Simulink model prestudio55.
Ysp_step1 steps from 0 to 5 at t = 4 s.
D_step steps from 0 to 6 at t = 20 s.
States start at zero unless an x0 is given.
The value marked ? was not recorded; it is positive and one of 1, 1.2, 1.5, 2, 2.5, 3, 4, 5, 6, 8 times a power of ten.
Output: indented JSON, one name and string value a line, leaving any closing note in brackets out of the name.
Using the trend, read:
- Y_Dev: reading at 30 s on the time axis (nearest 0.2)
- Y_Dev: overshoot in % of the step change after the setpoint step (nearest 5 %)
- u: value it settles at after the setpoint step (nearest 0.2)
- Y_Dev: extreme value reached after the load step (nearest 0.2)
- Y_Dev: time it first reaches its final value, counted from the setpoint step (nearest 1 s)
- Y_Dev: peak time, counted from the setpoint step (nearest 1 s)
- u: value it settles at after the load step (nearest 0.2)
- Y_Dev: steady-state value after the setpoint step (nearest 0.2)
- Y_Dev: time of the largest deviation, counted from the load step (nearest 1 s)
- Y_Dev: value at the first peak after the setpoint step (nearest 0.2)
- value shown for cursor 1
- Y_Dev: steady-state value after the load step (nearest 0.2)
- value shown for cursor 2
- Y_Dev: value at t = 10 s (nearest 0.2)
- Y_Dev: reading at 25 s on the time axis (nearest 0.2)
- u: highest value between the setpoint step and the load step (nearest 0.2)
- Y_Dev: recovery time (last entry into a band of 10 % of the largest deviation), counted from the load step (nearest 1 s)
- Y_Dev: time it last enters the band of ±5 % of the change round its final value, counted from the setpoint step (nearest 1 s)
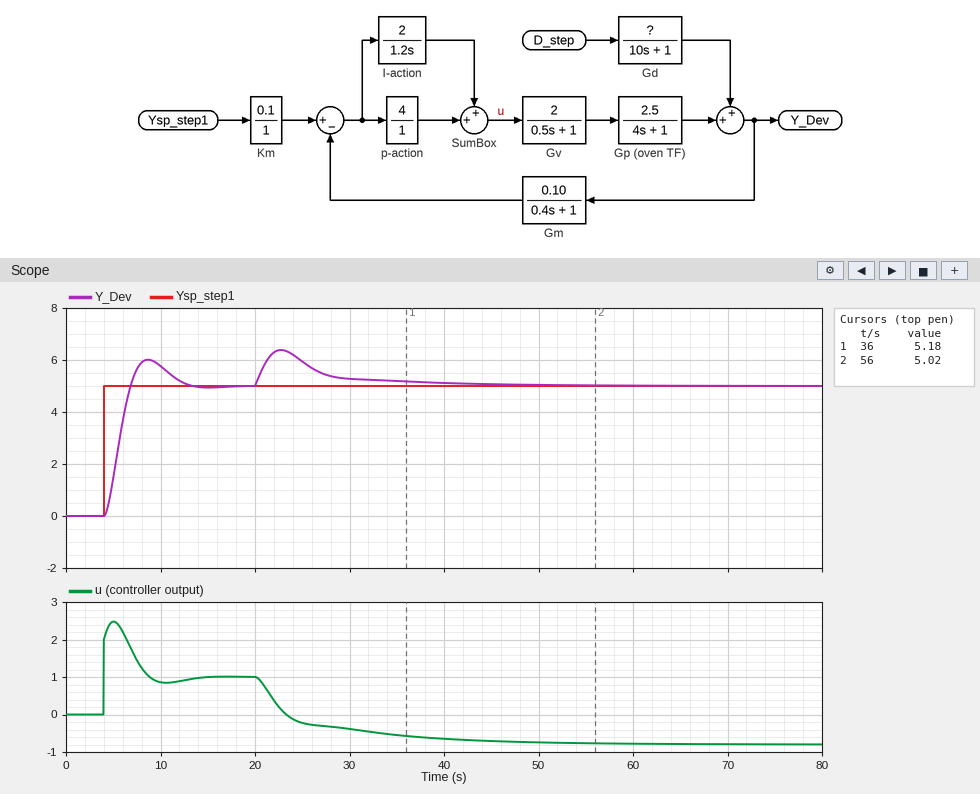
{
  "Y_Dev: reading at 30 s on the time axis": "5.2",
  "Y_Dev: overshoot in % of the step change after the setpoint step": "20 %",
  "u: value it settles at after the setpoint step": "1.0",
  "Y_Dev: extreme value reached after the load step": "6.4",
  "Y_Dev: time it first reaches its final value, counted from the setpoint step": "3 s",
  "Y_Dev: peak time, counted from the setpoint step": "5 s",
  "u: value it settles at after the load step": "-0.8",
  "Y_Dev: steady-state value after the setpoint step": "5.0",
  "Y_Dev: time of the largest deviation, counted from the load step": "3 s",
  "Y_Dev: value at the first peak after the setpoint step": "6.0",
  "value shown for cursor 1": "5.18",
  "Y_Dev: steady-state value after the load step": "5.0",
  "value shown for cursor 2": "5.02",
  "Y_Dev: value at t = 10 s": "5.8",
  "Y_Dev: reading at 25 s on the time axis": "6.0",
  "u: highest value between the setpoint step and the load step": "2.4",
  "Y_Dev: recovery time (last entry into a band of 10 % of the largest deviation), counted from the load step": "18 s",
  "Y_Dev: time it last enters the band of ±5 % of the change round its final value, counted from the setpoint step": "8 s"
}
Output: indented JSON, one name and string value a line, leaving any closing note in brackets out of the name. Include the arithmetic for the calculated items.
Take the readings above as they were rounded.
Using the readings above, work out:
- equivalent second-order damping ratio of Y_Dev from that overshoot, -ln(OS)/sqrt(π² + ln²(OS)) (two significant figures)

{
  "equivalent second-order damping ratio of Y_Dev from that overshoot, -ln(OS)/sqrt(π² + ln²(OS))": "ln(0.2) = -1.609; 1.609 / sqrt(9.870 + 2.590) = 0.46"
}
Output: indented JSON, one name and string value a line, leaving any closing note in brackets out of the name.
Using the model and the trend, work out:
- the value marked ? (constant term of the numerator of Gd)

{
  "the value marked ?": "1.5"
}
